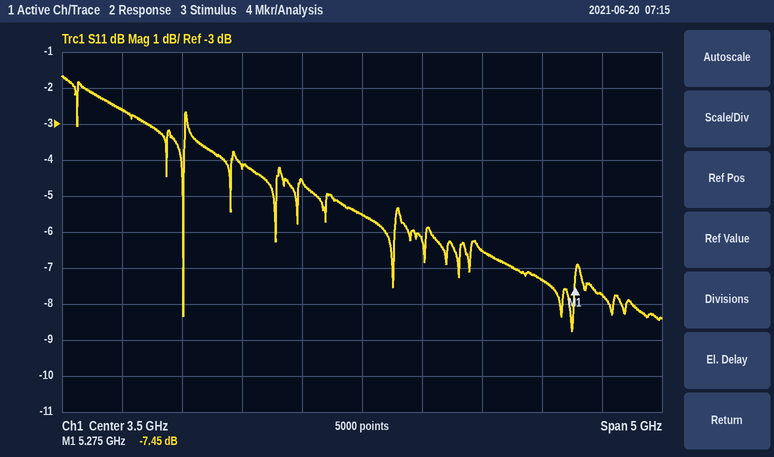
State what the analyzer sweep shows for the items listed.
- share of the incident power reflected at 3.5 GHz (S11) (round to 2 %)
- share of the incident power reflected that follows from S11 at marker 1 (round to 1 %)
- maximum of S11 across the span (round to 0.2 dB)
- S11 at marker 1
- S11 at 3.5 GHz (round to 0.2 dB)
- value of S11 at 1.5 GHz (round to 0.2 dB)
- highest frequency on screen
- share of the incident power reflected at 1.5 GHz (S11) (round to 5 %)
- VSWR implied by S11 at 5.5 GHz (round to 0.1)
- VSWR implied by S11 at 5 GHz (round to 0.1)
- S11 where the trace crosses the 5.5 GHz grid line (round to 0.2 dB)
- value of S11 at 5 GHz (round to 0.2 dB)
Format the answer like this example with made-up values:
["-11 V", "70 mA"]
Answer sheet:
["28 %", "18 %", "-1.6 dB", "-7.45 dB", "-5.6 dB", "-2.6 dB", "6 GHz", "55 %", "2.4", "2.5", "-7.8 dB", "-7.4 dB"]
